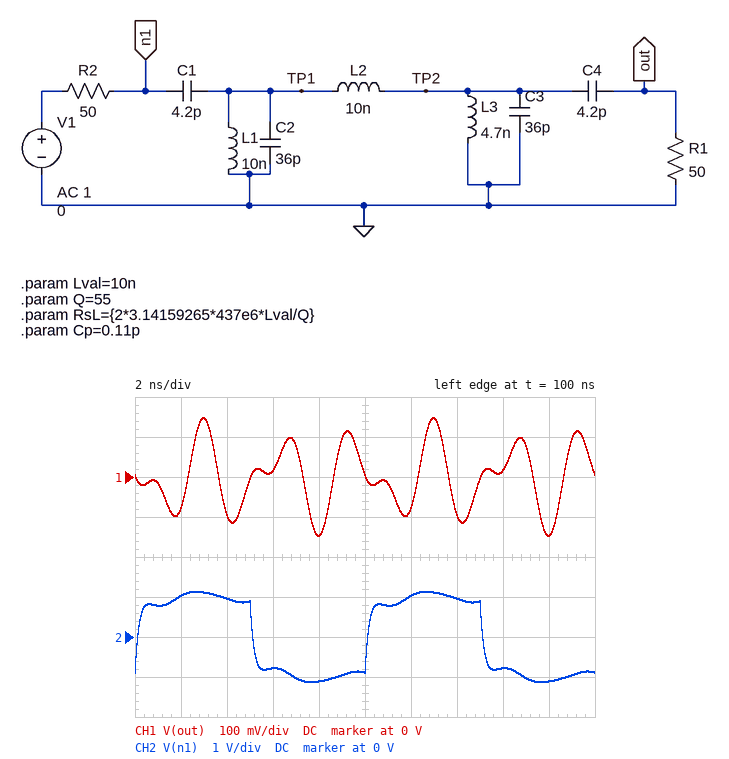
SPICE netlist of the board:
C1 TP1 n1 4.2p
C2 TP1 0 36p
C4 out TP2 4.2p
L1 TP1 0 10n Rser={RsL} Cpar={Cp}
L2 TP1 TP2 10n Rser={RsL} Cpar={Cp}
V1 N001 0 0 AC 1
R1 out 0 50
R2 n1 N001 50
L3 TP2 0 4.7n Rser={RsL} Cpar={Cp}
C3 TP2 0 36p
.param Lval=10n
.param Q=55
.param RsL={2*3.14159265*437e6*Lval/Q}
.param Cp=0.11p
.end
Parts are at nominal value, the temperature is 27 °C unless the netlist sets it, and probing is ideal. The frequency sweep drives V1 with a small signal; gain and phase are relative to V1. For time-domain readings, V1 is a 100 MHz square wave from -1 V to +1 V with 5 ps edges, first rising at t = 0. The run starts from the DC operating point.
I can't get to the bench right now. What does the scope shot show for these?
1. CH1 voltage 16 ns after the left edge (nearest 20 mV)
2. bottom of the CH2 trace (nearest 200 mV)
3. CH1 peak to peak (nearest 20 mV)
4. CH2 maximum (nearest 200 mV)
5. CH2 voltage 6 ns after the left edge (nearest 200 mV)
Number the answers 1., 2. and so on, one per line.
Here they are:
1. 20 mV
2. -1.2 V
3. 300 mV
4. 1.2 V
5. -800 mV
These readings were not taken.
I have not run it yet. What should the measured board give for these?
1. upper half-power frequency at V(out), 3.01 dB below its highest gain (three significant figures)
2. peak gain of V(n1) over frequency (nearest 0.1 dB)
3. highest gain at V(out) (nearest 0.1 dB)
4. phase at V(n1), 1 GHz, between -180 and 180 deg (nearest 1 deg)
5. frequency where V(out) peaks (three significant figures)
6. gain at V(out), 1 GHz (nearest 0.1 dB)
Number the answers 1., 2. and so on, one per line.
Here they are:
1. 505 MHz
2. 0 dB
3. -10.7 dB
4. -49 deg
5. 488 MHz
6. -46.0 dB
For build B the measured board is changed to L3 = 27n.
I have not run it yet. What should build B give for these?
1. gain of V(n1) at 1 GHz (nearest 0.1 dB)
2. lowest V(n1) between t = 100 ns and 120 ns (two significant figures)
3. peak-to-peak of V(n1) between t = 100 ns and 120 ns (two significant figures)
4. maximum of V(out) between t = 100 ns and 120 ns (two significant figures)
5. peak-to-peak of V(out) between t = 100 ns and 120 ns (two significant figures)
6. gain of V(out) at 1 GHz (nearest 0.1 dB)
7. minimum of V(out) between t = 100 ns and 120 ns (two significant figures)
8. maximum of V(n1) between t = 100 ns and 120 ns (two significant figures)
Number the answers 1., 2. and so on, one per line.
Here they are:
1. -3.7 dB
2. -1.0 V
3. 2.1 V
4. 33 mV
5. 66 mV
6. -47.2 dB
7. -33 mV
8. 1.0 V
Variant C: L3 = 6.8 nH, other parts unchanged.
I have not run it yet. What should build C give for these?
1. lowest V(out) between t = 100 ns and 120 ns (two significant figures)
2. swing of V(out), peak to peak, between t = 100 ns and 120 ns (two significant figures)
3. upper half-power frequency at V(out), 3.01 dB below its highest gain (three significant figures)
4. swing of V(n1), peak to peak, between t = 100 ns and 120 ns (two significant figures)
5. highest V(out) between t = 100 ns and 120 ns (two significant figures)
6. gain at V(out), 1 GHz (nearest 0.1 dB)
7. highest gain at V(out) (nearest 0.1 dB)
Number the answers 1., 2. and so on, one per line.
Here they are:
1. -73 mV
2. 150 mV
3. 472 MHz
4. 2.1 V
5. 73 mV
6. -46.4 dB
7. -9.3 dB
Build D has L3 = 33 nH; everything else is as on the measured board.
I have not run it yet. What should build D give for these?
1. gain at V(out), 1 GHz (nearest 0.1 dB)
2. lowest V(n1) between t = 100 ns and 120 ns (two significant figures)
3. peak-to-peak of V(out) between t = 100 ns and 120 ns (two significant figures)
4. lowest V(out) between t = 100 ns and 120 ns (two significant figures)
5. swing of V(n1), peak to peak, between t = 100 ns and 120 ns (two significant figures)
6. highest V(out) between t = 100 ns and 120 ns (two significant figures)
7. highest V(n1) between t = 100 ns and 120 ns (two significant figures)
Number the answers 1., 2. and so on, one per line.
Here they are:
1. -47.2 dB
2. -1.0 V
3. 64 mV
4. -32 mV
5. 2.1 V
6. 32 mV
7. 1.0 V
